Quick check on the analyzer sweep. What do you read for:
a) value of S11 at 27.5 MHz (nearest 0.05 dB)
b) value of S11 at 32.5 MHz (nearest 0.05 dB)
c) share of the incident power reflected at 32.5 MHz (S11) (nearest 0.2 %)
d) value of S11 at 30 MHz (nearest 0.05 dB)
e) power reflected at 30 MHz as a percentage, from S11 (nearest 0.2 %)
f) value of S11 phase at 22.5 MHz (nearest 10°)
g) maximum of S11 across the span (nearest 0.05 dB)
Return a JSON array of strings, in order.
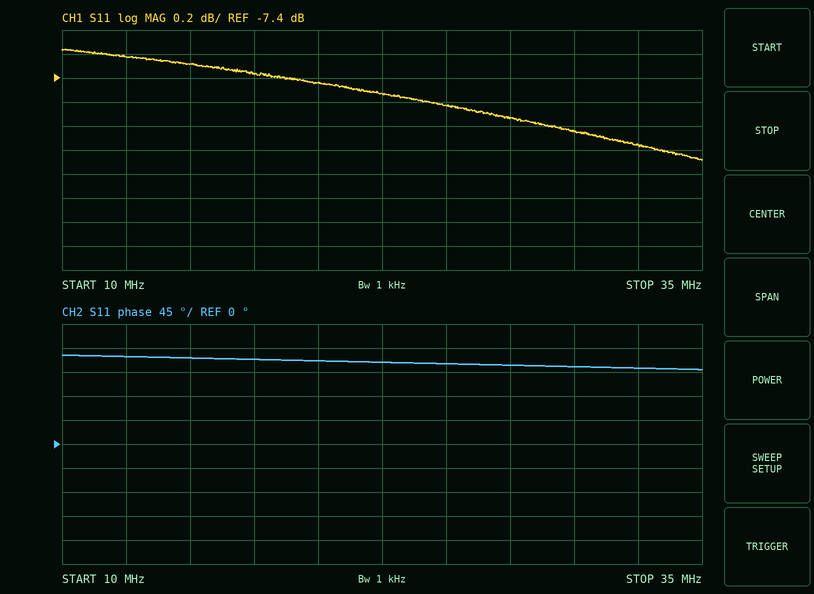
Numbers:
["-7.75 dB", "-7.95 dB", "16.0 %", "-7.85 dB", "16.4 %", "150°", "-7.15 dB"]
